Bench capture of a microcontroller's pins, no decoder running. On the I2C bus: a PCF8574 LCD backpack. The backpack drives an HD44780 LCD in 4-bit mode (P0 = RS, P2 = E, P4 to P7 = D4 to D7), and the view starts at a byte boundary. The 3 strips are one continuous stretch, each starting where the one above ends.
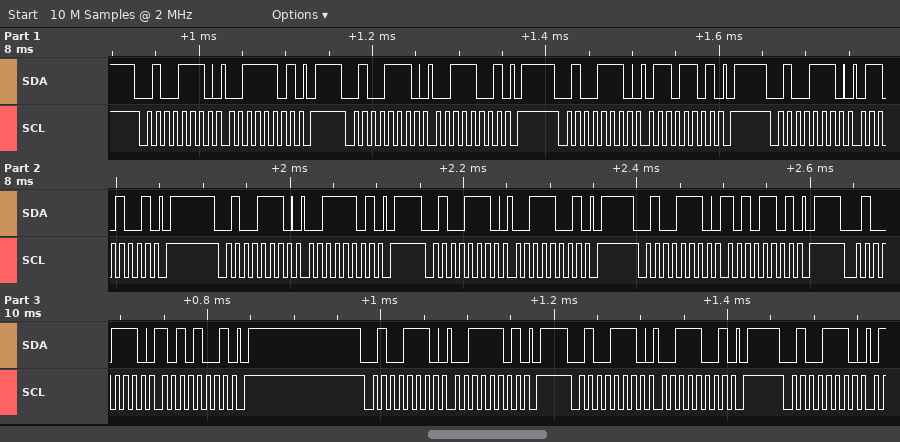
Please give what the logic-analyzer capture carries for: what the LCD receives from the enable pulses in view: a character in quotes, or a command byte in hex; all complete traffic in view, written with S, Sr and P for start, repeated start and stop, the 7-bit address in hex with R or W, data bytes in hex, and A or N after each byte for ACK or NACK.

'6' ':'
S 27W A 3D A P S 27W A 39 A P S 27W A 6D A P S 27W A 69 A P S 27W A 3D A P S 27W A 39 A P S 27W A AD A P S 27W A A9 A P S 27W A 3D A P S 27W A 39 A P S 27W A
